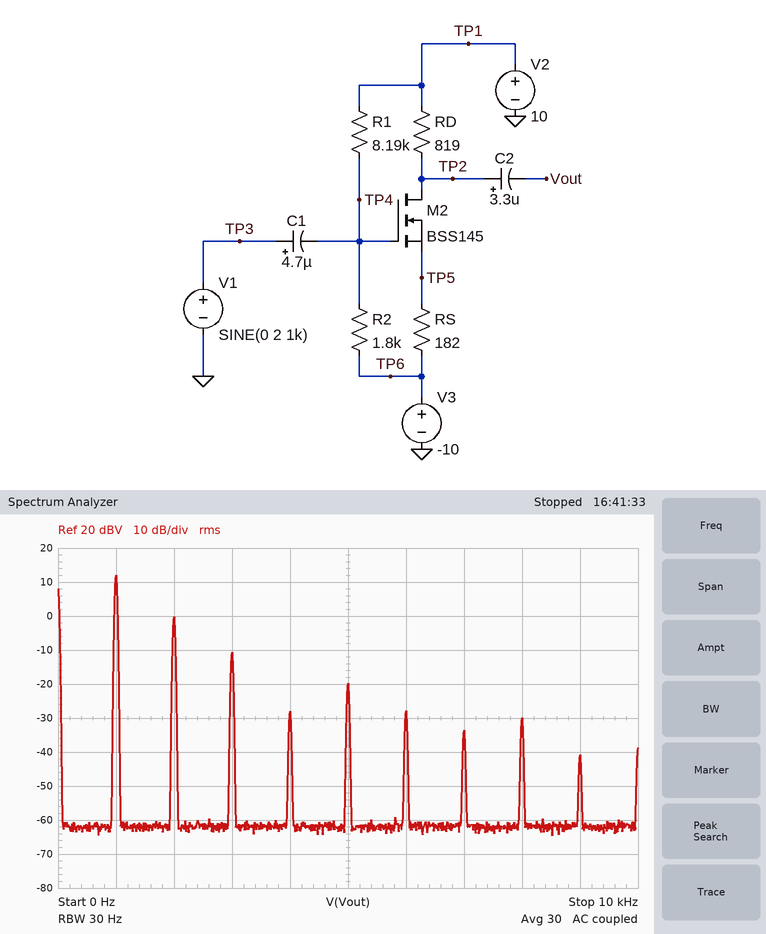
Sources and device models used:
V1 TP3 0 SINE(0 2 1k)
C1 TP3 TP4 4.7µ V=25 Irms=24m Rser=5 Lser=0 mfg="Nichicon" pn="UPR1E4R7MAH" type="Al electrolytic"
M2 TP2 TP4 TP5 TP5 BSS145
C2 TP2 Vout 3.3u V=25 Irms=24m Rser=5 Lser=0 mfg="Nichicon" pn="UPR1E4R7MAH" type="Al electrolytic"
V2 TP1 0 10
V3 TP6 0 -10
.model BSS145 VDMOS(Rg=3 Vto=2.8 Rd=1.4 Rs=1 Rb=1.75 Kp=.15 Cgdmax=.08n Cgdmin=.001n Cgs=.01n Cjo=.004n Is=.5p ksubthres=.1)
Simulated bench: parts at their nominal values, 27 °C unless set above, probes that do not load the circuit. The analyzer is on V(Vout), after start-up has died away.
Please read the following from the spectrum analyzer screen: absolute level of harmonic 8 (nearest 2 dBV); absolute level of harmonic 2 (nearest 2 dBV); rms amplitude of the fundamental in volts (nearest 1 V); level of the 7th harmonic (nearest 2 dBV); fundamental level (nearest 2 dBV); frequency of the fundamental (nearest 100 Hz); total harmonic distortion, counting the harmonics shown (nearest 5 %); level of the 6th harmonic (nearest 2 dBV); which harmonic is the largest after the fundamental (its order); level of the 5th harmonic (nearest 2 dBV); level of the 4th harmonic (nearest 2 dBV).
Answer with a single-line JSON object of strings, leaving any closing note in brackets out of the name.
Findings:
{"absolute level of harmonic 8": "-30 dBV", "absolute level of harmonic 2": "0 dBV", "rms amplitude of the fundamental in volts": "4 V", "level of the 7th harmonic": "-34 dBV", "fundamental level": "12 dBV", "frequency of the fundamental": "1.0 kHz", "total harmonic distortion, counting the harmonics shown": "25 %", "level of the 6th harmonic": "-28 dBV", "which harmonic is the largest after the fundamental": "2", "level of the 5th harmonic": "-20 dBV", "level of the 4th harmonic": "-28 dBV"}
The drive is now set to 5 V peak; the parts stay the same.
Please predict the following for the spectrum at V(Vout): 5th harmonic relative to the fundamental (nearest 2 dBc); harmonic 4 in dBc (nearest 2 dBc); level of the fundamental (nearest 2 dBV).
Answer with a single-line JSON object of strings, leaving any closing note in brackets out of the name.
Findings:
{"5th harmonic relative to the fundamental": "-36 dBc", "harmonic 4 in dBc": "-18 dBc", "level of the fundamental": "16 dBV"}
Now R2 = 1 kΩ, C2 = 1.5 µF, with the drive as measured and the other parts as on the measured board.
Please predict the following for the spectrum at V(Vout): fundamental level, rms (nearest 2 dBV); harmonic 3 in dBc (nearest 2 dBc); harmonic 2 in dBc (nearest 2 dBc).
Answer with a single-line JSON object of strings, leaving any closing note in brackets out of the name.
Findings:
{"fundamental level, rms": "4 dBV", "harmonic 3 in dBc": "-14 dBc", "harmonic 2 in dBc": "-4 dBc"}
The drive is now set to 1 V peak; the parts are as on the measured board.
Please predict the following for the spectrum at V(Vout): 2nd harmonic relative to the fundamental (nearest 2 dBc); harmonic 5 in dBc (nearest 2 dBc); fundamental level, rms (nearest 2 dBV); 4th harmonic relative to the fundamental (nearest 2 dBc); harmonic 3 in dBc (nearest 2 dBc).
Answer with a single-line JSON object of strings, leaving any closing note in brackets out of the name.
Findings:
{"2nd harmonic relative to the fundamental": "-22 dBc", "harmonic 5 in dBc": "-46 dBc", "fundamental level, rms": "8 dBV", "4th harmonic relative to the fundamental": "-36 dBc", "harmonic 3 in dBc": "-28 dBc"}
